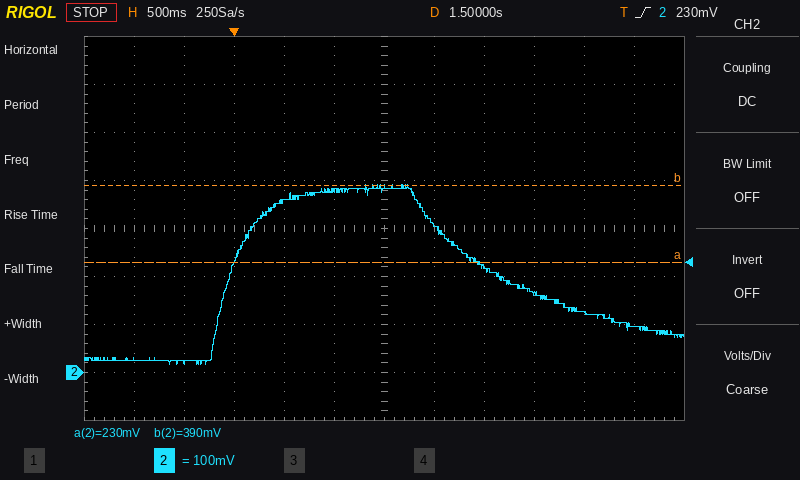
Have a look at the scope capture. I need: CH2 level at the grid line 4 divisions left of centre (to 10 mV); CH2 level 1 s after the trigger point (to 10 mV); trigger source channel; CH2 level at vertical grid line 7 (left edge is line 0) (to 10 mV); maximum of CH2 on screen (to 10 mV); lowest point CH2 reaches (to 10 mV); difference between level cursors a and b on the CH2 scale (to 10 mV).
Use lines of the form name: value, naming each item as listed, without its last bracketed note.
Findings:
CH2 level at the grid line 4 divisions left of centre: 20 mV
CH2 level 1 s after the trigger point: 380 mV
trigger source channel: CH2
CH2 level at vertical grid line 7 (left edge is line 0): 310 mV
maximum of CH2 on screen: 390 mV
lowest point CH2 reaches: 20 mV
difference between level cursors a and b on the CH2 scale: 160 mV
